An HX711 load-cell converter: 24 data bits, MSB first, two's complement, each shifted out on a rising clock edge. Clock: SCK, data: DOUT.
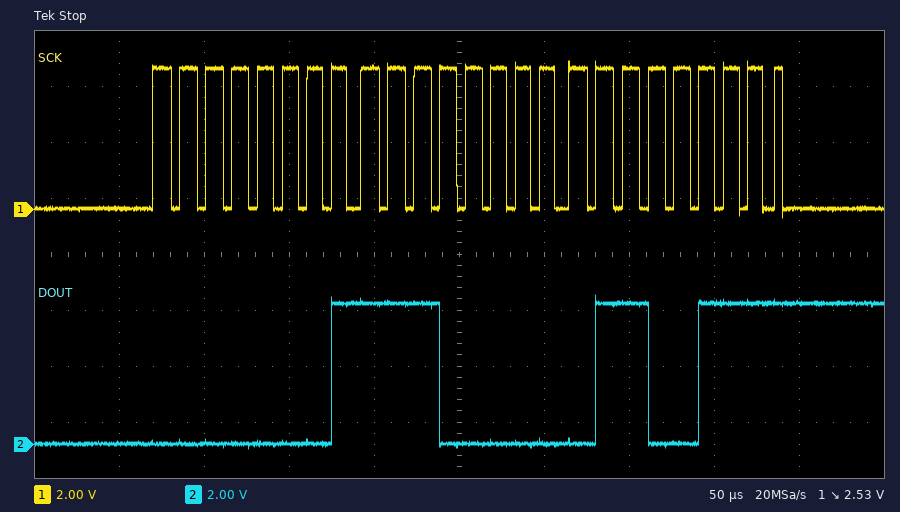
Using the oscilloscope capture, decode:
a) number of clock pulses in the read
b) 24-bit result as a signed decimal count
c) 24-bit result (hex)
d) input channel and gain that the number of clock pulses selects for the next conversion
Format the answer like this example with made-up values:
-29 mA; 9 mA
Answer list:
25; 122983; 0x01E067; channel A, gain 128
